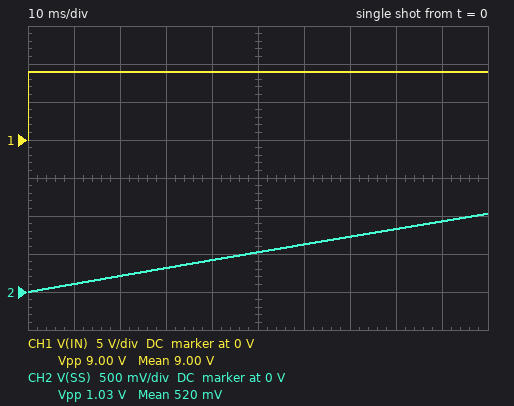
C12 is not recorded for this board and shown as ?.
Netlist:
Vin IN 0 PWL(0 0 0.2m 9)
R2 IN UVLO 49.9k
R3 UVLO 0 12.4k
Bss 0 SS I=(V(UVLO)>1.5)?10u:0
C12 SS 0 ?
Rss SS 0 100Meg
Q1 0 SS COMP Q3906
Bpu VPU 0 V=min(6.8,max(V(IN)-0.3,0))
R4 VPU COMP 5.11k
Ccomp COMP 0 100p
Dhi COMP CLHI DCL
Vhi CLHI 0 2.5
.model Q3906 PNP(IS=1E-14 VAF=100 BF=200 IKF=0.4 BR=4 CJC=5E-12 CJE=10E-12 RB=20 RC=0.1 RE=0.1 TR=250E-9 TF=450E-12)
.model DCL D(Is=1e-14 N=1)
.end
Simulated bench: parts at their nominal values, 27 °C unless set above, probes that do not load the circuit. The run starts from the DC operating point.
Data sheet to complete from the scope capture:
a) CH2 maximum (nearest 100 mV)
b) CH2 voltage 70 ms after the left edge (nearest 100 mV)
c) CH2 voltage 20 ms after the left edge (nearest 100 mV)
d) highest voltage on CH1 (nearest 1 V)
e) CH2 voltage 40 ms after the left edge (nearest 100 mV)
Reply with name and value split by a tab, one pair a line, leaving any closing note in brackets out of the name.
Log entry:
CH2 maximum	1.0 V
CH2 voltage 70 ms after the left edge	700 mV
CH2 voltage 20 ms after the left edge	200 mV
highest voltage on CH1	9 V
CH2 voltage 40 ms after the left edge	400 mV
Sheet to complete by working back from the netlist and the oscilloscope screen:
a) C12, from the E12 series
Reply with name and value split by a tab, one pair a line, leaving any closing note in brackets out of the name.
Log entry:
C12, from the E12 series	1.5 µF
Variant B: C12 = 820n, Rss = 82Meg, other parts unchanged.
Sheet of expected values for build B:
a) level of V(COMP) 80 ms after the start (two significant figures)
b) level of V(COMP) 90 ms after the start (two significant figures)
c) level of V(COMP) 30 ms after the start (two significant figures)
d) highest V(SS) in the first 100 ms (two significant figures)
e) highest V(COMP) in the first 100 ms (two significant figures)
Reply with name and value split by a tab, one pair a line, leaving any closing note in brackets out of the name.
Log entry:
level of V(COMP) 80 ms after the start	2.1 V
level of V(COMP) 90 ms after the start	2.3 V
level of V(COMP) 30 ms after the start	1.2 V
highest V(SS) in the first 100 ms	1.8 V
highest V(COMP) in the first 100 ms	2.5 V
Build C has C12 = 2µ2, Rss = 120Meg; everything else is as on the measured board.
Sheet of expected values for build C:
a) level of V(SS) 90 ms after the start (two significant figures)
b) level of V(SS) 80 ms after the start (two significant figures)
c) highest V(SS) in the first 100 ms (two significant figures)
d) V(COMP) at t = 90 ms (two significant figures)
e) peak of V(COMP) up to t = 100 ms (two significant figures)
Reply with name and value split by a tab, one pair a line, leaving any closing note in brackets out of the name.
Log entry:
level of V(SS) 90 ms after the start	640 mV
level of V(SS) 80 ms after the start	570 mV
highest V(SS) in the first 100 ms	710 mV
V(COMP) at t = 90 ms	1.3 V
peak of V(COMP) up to t = 100 ms	1.4 V
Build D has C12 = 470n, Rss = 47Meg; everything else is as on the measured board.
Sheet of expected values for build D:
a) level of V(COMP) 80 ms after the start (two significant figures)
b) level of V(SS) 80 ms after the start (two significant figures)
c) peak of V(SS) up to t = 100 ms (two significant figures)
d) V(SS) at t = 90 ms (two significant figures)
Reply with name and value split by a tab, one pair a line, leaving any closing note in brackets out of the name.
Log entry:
level of V(COMP) 80 ms after the start	3.1 V
level of V(SS) 80 ms after the start	2.5 V
peak of V(SS) up to t = 100 ms	2.9 V
V(SS) at t = 90 ms	2.7 V
